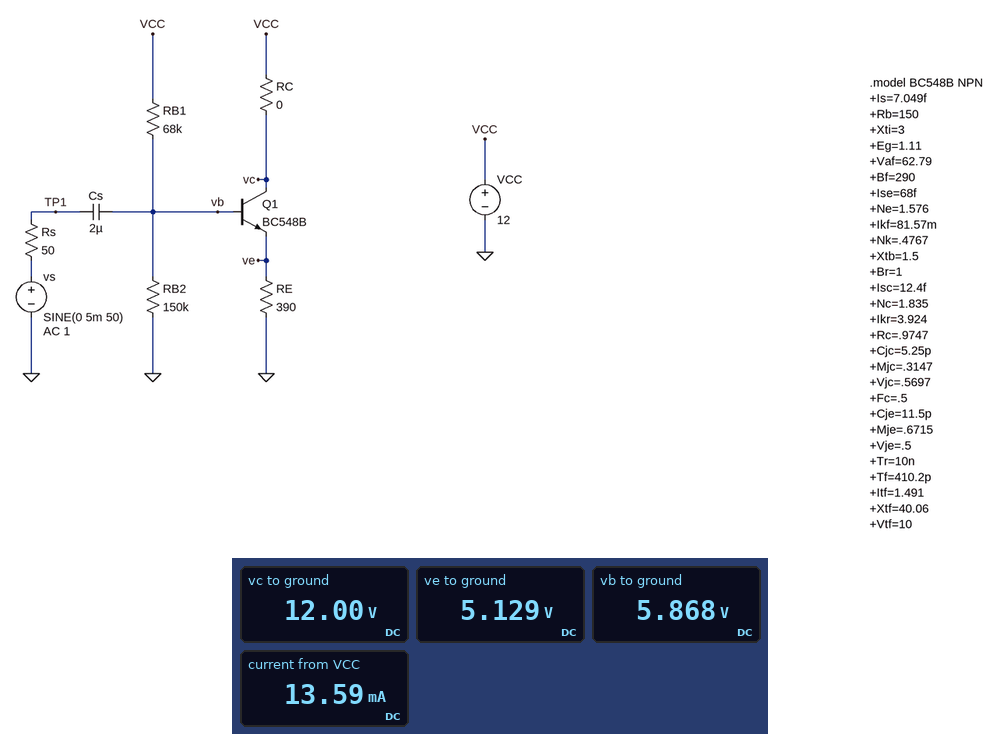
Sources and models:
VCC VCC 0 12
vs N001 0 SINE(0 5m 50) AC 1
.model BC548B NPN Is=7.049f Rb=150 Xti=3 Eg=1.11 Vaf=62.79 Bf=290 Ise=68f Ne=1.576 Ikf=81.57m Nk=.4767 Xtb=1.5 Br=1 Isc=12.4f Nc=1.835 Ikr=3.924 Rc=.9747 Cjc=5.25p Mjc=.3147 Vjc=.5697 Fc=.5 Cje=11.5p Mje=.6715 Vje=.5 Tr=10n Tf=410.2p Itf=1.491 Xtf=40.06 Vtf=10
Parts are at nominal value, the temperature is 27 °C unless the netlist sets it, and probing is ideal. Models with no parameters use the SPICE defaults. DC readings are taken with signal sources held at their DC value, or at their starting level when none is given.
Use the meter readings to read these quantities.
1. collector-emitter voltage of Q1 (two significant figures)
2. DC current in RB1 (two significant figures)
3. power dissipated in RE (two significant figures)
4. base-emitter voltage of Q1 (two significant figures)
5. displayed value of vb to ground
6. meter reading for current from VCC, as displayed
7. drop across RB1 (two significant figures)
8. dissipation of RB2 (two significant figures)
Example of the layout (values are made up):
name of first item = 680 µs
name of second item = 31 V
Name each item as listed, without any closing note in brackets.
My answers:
collector-emitter voltage of Q1 = 6.9 V
DC current in RB1 = 90 µA
power dissipated in RE = 67 mW
base-emitter voltage of Q1 = 740 mV
displayed value of vb to ground = 5.868 V
meter reading for current from VCC, as displayed = 13.59 mA
drop across RB1 = 6.1 V
dissipation of RB2 = 230 µW
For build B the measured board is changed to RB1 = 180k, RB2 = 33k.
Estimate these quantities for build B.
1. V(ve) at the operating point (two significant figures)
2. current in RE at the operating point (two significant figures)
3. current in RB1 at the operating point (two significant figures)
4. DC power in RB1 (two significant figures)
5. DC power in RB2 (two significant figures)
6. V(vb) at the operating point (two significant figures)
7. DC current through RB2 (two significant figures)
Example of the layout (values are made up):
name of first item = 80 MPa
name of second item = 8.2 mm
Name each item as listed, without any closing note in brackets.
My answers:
V(ve) at the operating point = 940 mV
current in RE at the operating point = 2.4 mA
current in RB1 at the operating point = 58 µA
DC power in RB1 = 600 µW
DC power in RB2 = 80 µW
V(vb) at the operating point = 1.6 V
DC current through RB2 = 49 µA
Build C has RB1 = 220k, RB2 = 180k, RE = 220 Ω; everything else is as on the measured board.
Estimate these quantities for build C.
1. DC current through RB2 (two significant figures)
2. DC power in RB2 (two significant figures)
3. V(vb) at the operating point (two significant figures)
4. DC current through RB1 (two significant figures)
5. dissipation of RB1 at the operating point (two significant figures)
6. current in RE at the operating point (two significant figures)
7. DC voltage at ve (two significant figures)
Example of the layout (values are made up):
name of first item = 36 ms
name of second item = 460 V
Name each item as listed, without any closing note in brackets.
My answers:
DC current through RB2 = 14 µA
DC power in RB2 = 35 µW
V(vb) at the operating point = 2.5 V
DC current through RB1 = 43 µA
dissipation of RB1 at the operating point = 410 µW
current in RE at the operating point = 8.1 mA
DC voltage at ve = 1.8 V
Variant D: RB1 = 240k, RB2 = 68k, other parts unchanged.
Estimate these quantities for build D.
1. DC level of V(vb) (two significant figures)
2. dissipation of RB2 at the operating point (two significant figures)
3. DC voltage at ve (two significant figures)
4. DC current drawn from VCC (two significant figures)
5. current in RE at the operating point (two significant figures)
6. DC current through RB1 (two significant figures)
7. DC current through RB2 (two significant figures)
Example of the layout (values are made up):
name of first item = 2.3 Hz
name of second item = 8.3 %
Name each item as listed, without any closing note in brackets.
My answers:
DC level of V(vb) = 2.0 V
dissipation of RB2 at the operating point = 60 µW
DC voltage at ve = 1.3 V
DC current drawn from VCC = 3.9 mA
current in RE at the operating point = 3.4 mA
DC current through RB1 = 42 µA
DC current through RB2 = 30 µA
